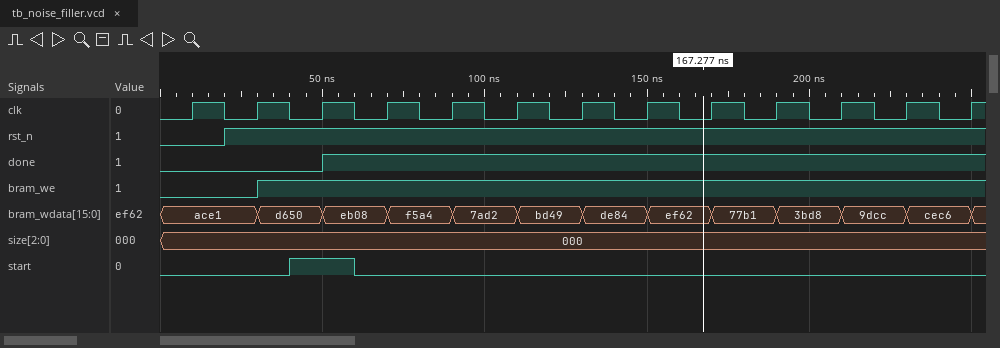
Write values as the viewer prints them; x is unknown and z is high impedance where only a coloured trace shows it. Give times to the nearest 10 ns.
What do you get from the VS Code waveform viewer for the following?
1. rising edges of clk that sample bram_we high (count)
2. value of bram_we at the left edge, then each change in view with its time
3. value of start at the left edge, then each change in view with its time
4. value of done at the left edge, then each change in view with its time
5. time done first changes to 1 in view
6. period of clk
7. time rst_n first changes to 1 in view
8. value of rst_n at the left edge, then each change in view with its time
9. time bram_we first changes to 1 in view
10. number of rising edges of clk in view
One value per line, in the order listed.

11
0, 1 at 30 ns
0, 1 at 40 ns, 0 at 60 ns
0, 1 at 50 ns
50 ns
20 ns
20 ns
0, 1 at 20 ns
30 ns
13
